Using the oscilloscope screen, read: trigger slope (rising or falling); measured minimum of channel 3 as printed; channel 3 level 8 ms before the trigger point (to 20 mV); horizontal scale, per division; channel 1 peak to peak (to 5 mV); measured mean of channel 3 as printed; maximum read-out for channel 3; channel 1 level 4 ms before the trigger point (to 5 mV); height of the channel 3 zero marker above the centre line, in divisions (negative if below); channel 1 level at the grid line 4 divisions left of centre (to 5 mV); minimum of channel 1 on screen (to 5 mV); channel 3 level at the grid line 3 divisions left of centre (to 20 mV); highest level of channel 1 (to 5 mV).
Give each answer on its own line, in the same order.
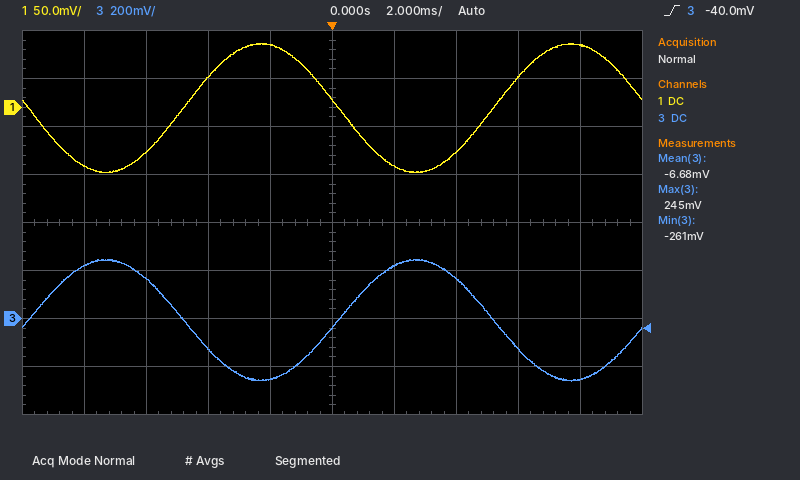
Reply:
rising
-261 mV
220 mV
2 ms
135 mV
-6.68 mV
245 mV
30 mV
-2.0 div
-60 mV
-70 mV
160 mV
65 mV
